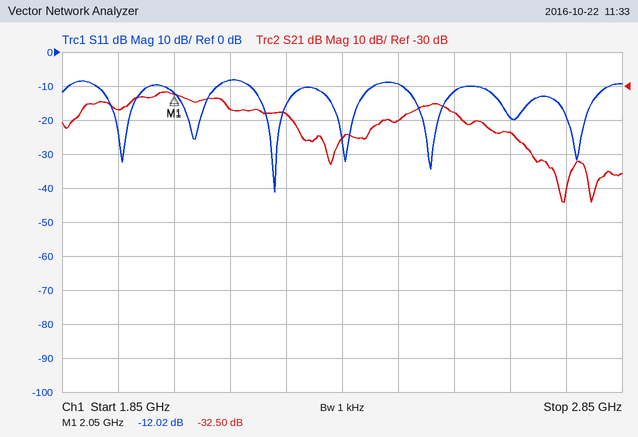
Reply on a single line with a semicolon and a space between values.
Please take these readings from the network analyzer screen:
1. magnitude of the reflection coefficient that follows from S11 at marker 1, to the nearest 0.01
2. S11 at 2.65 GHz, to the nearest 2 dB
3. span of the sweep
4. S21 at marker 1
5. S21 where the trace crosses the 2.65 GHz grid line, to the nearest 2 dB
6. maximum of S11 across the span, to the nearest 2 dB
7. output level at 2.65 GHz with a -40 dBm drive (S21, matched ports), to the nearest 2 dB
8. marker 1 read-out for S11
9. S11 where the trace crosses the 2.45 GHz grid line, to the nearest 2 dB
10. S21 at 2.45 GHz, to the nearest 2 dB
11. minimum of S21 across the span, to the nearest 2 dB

0.25; -20 dB; 1 GHz; -32.50 dB; -44 dB; -8 dB; -84 dBm; -12.02 dB; -10 dB; -40 dB; -64 dB
